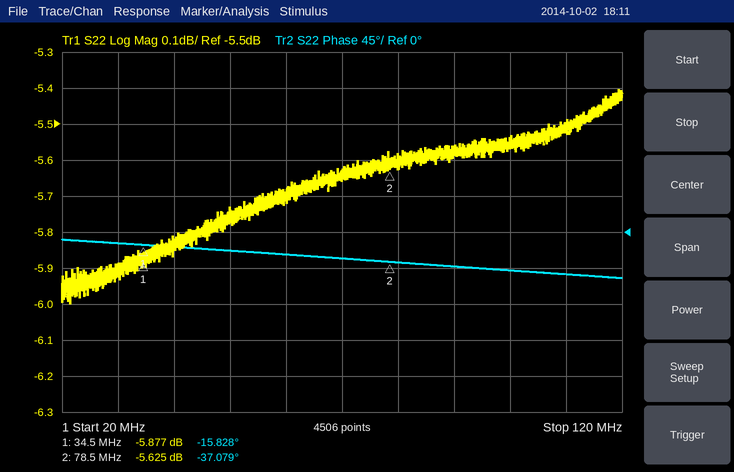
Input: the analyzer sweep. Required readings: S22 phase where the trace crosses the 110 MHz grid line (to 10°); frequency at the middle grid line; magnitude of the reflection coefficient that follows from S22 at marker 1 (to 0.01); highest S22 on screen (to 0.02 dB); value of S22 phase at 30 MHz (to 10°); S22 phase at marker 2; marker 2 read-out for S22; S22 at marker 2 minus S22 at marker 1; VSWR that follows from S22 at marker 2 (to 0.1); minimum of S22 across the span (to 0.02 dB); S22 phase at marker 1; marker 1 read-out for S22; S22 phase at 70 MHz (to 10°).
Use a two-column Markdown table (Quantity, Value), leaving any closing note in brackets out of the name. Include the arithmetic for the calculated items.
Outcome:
| Quantity | Value |
|---|---|
| S22 phase where the trace crosses the 110 MHz grid line | -50° |
| frequency at the middle grid line | 70 MHz |
| magnitude of the reflection coefficient that follows from S22 at marker 1 | 10^(-5.877/20) ≈ 0.51 |
| highest S22 on screen | -5.40 dB |
| value of S22 phase at 30 MHz | -10° |
| S22 phase at marker 2 | -37.079° |
| marker 2 read-out for S22 | -5.625 dB |
| S22 at marker 2 minus S22 at marker 1 | -5.625 − (-5.877) = 0.252 dB |
| VSWR that follows from S22 at marker 2 | (1 + 0.5233)/(1 − 0.5233) ≈ 3.2 |
| minimum of S22 across the span | -6.00 dB |
| S22 phase at marker 1 | -15.828° |
| marker 1 read-out for S22 | -5.877 dB |
| S22 phase at 70 MHz | -30° |
